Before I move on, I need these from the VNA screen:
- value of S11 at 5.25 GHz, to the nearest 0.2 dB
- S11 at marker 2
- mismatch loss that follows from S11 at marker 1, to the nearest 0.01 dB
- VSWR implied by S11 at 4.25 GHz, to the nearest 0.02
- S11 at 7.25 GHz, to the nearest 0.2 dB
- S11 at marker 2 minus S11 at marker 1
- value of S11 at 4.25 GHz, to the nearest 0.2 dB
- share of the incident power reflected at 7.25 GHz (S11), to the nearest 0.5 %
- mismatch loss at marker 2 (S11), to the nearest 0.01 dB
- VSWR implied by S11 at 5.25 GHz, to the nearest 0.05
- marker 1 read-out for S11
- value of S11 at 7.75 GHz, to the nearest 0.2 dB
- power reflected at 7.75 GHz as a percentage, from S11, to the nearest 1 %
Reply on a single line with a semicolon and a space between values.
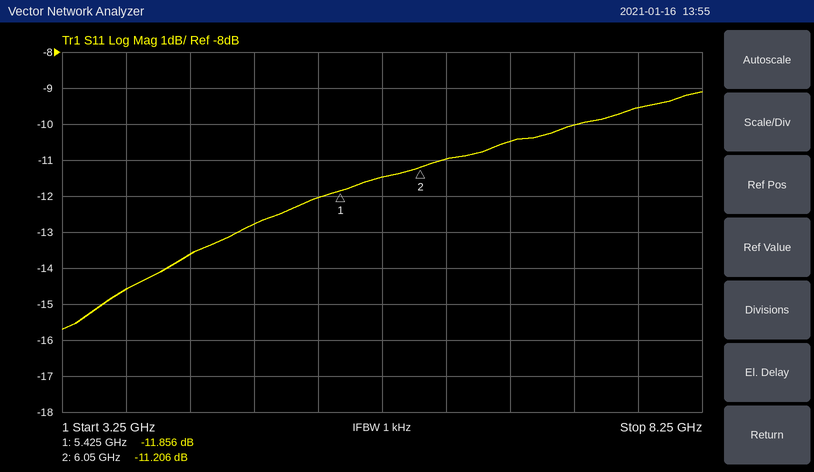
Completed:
-12.0 dB; -11.206 dB; 0.29 dB; 1.52; -10.0 dB; 0.650 dB; -13.6 dB; 10.0 %; 0.34 dB; 1.65; -11.856 dB; -9.6 dB; 11 %
